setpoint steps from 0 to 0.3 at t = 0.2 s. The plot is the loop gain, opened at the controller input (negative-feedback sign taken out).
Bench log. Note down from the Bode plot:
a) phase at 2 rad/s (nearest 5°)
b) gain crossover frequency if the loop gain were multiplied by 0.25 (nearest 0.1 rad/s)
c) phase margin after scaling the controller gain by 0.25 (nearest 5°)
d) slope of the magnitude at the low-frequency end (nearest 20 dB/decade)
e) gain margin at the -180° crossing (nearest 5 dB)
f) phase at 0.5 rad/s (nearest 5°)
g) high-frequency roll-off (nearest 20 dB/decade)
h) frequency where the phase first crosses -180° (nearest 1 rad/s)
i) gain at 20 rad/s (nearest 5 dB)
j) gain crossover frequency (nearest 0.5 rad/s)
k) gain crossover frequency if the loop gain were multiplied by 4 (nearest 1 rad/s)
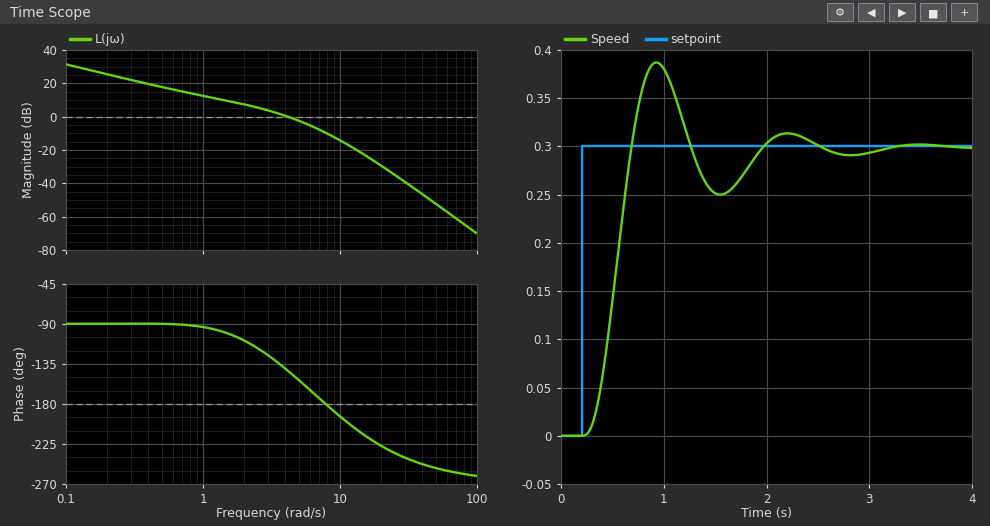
-110°
1.1 rad/s
85°
-20 dB/decade
10 dB
-90°
-60 dB/decade
8 rad/s
-30 dB
4.0 rad/s
9 rad/s
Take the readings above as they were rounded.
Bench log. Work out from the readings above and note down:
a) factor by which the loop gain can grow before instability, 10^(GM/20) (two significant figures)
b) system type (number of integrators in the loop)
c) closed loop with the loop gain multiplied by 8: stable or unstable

3.2
1
unstable
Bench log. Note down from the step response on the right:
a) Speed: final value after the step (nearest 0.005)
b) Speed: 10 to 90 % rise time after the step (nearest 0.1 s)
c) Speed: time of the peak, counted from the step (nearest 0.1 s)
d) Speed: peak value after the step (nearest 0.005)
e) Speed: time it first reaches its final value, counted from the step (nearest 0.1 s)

0.300
0.3 s
0.7 s
0.385
0.5 s
